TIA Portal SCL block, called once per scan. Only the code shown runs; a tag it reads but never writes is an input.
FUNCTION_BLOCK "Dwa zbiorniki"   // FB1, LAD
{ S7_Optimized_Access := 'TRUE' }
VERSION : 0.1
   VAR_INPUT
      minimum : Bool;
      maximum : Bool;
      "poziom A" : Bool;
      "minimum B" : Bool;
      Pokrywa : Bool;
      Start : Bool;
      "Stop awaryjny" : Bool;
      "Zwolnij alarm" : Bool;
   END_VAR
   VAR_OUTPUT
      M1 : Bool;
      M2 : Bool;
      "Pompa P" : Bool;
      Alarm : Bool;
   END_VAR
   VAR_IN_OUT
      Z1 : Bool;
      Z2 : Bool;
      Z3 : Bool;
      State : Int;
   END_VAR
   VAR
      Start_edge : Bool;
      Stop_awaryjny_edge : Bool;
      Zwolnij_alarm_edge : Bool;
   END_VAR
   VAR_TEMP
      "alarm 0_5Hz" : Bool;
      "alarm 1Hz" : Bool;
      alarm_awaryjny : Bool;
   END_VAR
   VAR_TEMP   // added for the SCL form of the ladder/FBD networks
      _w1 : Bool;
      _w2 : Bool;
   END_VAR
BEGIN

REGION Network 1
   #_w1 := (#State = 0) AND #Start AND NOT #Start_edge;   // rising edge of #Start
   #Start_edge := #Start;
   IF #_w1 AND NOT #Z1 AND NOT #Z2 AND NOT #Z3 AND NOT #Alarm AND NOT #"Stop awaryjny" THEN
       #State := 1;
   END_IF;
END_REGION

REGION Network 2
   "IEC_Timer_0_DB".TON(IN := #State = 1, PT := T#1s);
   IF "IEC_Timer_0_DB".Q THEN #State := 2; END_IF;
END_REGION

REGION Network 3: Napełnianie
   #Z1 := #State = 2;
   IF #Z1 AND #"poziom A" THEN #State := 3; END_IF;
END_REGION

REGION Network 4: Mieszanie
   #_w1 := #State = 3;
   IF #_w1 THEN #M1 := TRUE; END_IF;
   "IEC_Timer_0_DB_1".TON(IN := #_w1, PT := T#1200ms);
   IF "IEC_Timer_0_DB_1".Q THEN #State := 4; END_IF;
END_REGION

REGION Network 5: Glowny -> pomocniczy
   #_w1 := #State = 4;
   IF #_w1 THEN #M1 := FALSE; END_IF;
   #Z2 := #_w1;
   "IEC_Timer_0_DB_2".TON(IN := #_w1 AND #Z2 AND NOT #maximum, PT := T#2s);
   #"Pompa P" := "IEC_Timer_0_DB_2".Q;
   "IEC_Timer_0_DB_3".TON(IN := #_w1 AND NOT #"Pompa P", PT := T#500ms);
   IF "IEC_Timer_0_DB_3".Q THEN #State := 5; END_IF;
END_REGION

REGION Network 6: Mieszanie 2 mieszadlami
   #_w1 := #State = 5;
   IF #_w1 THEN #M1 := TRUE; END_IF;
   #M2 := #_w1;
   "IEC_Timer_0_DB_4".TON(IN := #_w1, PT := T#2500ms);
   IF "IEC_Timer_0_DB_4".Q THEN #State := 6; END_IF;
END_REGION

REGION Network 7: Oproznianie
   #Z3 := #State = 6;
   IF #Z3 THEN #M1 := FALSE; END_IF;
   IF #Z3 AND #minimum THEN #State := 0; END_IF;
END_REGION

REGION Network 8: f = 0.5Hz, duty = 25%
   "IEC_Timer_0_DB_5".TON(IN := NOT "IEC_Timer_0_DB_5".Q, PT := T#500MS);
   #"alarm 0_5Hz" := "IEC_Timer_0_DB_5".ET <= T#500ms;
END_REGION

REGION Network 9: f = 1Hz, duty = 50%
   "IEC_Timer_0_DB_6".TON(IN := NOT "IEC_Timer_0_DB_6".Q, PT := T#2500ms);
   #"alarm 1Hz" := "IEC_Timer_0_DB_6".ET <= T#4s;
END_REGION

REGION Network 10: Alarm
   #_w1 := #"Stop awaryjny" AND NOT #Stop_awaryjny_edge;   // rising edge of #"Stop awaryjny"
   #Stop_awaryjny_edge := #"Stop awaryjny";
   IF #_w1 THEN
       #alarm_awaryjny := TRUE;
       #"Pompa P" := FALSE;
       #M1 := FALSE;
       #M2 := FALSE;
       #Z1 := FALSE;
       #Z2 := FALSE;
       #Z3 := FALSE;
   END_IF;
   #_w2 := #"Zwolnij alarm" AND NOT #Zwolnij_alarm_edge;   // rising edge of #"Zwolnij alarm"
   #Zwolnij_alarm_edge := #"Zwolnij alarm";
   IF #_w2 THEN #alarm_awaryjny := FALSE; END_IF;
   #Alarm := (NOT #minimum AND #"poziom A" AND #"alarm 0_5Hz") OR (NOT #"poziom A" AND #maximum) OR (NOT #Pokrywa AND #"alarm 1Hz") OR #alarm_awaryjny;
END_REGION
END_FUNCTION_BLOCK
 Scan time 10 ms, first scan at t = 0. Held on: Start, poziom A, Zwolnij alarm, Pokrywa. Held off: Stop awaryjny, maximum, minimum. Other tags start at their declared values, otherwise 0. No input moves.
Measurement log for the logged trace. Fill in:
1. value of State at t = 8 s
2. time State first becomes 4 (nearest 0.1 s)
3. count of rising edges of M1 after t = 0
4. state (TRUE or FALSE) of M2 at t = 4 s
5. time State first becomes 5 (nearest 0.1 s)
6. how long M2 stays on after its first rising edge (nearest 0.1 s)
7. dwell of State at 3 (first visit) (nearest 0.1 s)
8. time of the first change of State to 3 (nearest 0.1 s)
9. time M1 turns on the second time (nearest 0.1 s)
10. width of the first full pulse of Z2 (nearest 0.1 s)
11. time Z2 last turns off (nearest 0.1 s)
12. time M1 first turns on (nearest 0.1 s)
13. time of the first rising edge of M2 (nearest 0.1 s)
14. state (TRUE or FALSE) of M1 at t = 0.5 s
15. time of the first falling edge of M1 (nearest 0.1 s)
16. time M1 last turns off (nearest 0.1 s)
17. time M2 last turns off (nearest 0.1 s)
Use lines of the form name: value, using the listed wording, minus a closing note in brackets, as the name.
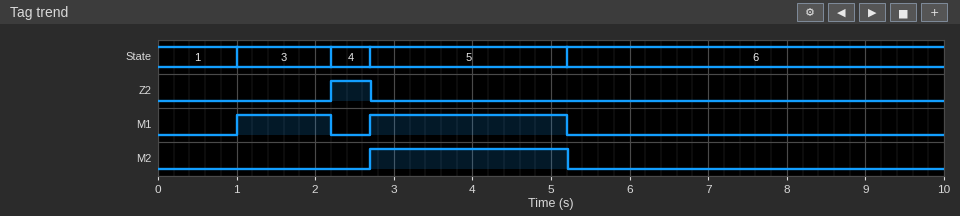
value of State at t = 8 s: 6
time State first becomes 4: 2.2 s
count of rising edges of M1 after t = 0: 2
state (TRUE or FALSE) of M2 at t = 4 s: TRUE
time State first becomes 5: 2.7 s
how long M2 stays on after its first rising edge: 2.5 s
dwell of State at 3 (first visit): 1.2 s
time of the first change of State to 3: 1.0 s
time M1 turns on the second time: 2.7 s
width of the first full pulse of Z2: 0.5 s
time Z2 last turns off: 2.7 s
time M1 first turns on: 1.0 s
time of the first rising edge of M2: 2.7 s
state (TRUE or FALSE) of M1 at t = 0.5 s: FALSE
time of the first falling edge of M1: 2.2 s
time M1 last turns off: 5.2 s
time M2 last turns off: 5.2 s
